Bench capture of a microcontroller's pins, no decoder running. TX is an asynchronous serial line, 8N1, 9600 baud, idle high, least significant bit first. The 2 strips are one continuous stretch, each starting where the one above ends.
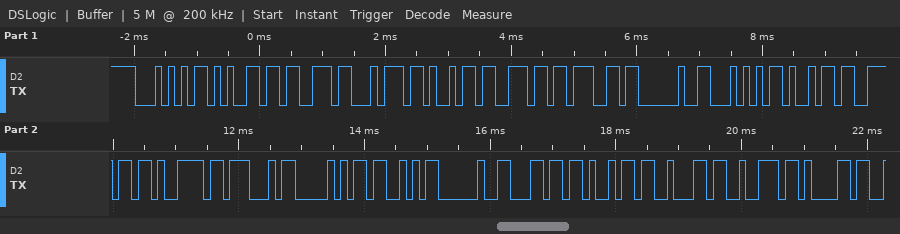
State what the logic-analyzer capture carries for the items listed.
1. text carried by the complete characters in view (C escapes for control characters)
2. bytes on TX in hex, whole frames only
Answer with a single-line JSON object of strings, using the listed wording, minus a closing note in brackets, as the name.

{"text carried by the complete characters in view": "\"Testing TinyGPS libra\"", "bytes on TX in hex, whole frames only": "0x54 0x65 0x73 0x74 0x69 0x6E 0x67 0x20 0x54 0x69 0x6E 0x79 0x47 0x50 0x53 0x20 0x6C 0x69 0x62 0x72 0x61"}
